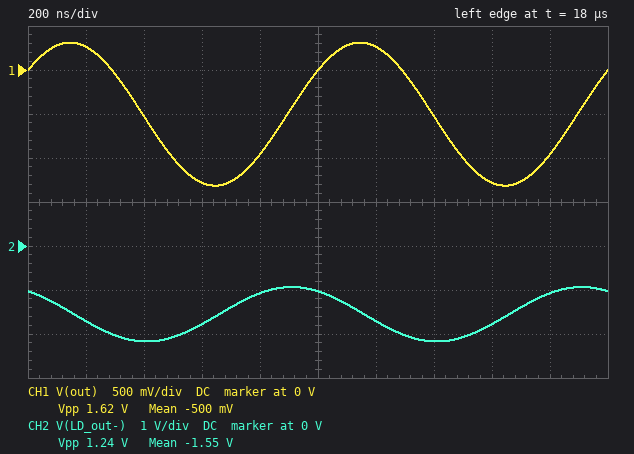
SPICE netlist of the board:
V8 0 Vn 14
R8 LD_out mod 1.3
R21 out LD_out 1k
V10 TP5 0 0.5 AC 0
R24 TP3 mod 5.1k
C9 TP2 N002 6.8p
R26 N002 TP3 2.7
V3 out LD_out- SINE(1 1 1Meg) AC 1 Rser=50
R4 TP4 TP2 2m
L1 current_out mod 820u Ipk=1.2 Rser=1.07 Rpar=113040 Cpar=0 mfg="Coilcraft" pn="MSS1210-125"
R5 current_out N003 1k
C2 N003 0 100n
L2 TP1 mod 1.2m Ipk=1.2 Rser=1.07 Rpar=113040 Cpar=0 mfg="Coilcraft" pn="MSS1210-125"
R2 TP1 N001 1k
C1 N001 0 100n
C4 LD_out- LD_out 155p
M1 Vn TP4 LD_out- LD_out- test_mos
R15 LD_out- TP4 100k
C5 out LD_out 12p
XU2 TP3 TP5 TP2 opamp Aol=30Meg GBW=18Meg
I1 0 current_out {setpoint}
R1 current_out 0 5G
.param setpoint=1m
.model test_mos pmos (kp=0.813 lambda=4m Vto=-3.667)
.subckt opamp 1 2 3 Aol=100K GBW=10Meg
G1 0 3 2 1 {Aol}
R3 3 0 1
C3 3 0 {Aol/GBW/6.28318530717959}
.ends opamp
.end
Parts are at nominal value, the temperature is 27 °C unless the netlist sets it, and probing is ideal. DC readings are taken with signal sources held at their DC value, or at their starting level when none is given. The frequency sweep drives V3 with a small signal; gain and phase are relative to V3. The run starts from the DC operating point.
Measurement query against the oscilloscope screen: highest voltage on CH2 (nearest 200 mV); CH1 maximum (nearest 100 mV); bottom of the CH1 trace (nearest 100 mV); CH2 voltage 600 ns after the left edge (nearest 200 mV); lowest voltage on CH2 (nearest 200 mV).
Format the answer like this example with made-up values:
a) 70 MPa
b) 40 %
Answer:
a) -1.0 V
b) 300 mV
c) -1.3 V
d) -1.8 V
e) -2.2 V
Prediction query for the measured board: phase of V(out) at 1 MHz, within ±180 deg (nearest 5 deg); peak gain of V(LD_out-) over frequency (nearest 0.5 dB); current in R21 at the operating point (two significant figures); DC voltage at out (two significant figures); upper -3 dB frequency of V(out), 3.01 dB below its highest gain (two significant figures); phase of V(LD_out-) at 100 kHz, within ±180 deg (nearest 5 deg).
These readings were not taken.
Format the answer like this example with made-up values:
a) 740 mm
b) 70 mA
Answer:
a) 40 deg
b) 0 dB
c) 1.0 mA
d) -500 mV
e) 250 MHz
f) 170 deg
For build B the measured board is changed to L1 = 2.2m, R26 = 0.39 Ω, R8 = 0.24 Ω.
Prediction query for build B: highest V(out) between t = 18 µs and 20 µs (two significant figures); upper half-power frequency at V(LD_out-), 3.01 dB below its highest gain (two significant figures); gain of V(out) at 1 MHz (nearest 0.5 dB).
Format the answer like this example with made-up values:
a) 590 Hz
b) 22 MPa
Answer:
a) 320 mV
b) 790 kHz
c) -1.5 dB
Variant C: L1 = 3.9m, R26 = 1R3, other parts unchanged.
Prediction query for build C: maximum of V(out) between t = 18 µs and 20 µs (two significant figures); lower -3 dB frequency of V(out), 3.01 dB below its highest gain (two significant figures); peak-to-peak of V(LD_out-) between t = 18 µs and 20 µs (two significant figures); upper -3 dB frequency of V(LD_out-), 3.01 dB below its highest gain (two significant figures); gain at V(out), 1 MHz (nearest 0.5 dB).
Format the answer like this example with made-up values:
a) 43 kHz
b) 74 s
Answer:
a) 320 mV
b) 790 kHz
c) 1.3 V
d) 800 kHz
e) -1.5 dB
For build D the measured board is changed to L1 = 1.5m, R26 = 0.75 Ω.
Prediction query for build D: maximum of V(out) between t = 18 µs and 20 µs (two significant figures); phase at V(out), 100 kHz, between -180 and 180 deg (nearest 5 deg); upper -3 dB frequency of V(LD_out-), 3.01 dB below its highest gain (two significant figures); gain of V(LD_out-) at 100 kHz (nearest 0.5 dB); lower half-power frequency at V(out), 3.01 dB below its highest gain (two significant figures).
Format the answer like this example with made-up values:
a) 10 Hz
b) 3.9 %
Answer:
a) 320 mV
b) 70 deg
c) 780 kHz
d) -0.5 dB
e) 800 kHz
